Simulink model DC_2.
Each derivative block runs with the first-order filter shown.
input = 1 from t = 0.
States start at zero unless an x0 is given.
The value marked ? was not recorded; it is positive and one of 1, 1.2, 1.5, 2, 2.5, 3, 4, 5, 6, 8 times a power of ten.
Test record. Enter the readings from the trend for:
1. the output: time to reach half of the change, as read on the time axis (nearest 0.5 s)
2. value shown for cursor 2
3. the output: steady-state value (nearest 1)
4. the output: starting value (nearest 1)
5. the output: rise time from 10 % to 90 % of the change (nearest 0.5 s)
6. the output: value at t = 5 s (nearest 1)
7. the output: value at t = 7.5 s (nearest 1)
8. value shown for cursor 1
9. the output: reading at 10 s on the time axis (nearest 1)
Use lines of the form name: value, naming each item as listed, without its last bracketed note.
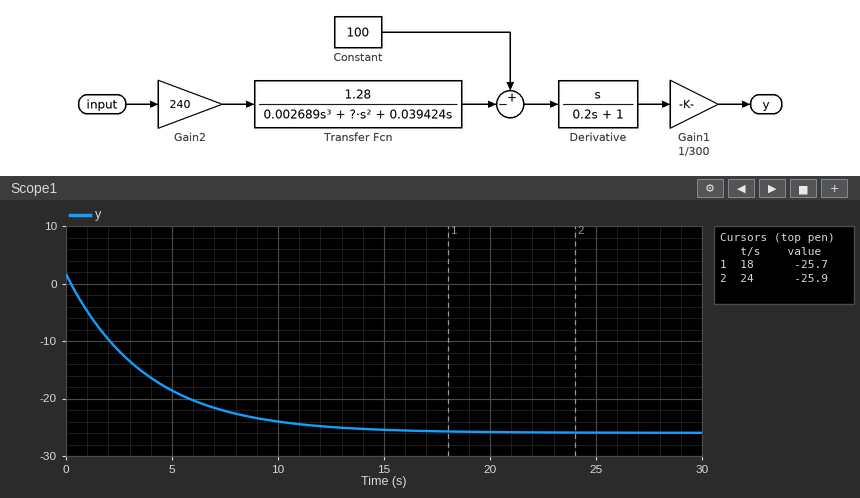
the output: time to reach half of the change, as read on the time axis: 2.5 s
value shown for cursor 2: -25.9
the output: steady-state value: -26
the output: starting value: 2
the output: rise time from 10 % to 90 % of the change: 8.5 s
the output: value at t = 5 s: -19
the output: value at t = 7.5 s: -22
value shown for cursor 1: -25.7
the output: reading at 10 s on the time axis: -24
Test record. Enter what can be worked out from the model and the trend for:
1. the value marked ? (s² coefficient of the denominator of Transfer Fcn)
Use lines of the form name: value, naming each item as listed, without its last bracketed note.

the value marked ?: 0.15
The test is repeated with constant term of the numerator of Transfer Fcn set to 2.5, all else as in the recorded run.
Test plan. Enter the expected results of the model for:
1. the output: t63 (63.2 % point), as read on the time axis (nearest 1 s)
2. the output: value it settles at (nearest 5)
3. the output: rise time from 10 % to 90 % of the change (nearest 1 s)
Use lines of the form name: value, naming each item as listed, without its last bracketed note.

the output: t63 (63.2 % point), as read on the time axis: 4 s
the output: value it settles at: -50
the output: rise time from 10 % to 90 % of the change: 8 s
